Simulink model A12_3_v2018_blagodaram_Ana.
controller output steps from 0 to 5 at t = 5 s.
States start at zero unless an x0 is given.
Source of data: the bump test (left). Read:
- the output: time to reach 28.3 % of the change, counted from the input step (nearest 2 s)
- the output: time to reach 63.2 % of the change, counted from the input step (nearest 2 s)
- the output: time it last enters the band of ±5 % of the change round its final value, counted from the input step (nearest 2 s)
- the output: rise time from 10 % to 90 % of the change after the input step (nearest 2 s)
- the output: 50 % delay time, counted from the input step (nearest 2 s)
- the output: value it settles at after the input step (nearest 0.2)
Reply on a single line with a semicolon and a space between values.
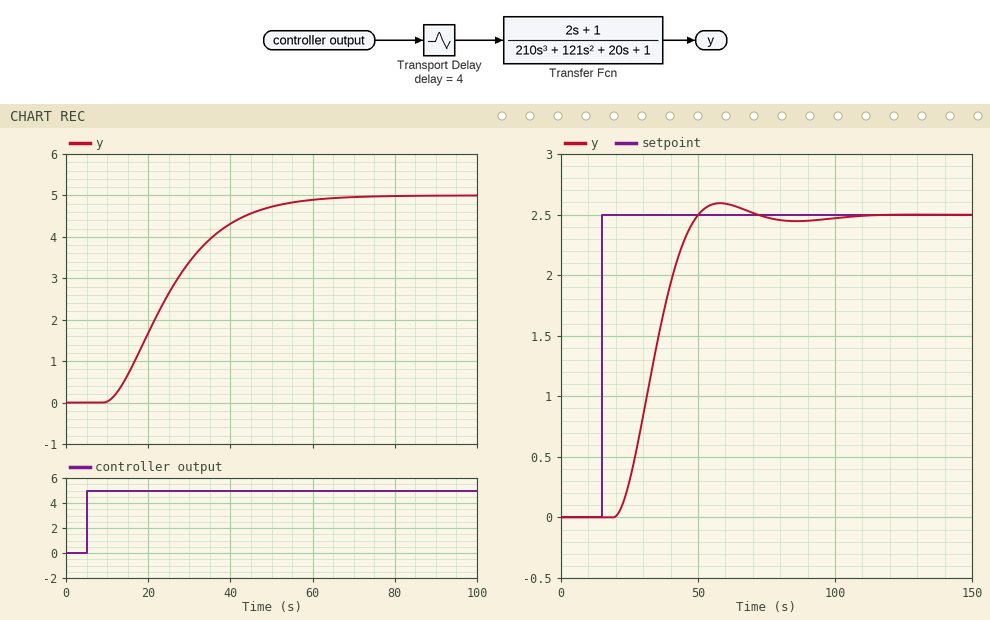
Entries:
14 s; 24 s; 46 s; 30 s; 20 s; 5.0
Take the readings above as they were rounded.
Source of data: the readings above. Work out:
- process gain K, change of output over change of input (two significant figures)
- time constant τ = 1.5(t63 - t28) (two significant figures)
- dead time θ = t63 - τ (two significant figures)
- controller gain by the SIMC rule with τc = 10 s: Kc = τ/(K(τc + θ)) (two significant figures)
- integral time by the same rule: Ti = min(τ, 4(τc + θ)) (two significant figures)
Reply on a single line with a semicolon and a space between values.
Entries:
1.0; 15 s; 9.0 s; 0.79; 15 s
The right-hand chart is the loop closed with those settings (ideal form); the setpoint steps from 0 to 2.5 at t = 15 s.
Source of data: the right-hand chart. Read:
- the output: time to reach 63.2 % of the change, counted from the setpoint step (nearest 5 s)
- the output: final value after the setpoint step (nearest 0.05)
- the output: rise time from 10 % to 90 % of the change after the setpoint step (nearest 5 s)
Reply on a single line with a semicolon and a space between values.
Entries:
20 s; 2.50; 20 s
